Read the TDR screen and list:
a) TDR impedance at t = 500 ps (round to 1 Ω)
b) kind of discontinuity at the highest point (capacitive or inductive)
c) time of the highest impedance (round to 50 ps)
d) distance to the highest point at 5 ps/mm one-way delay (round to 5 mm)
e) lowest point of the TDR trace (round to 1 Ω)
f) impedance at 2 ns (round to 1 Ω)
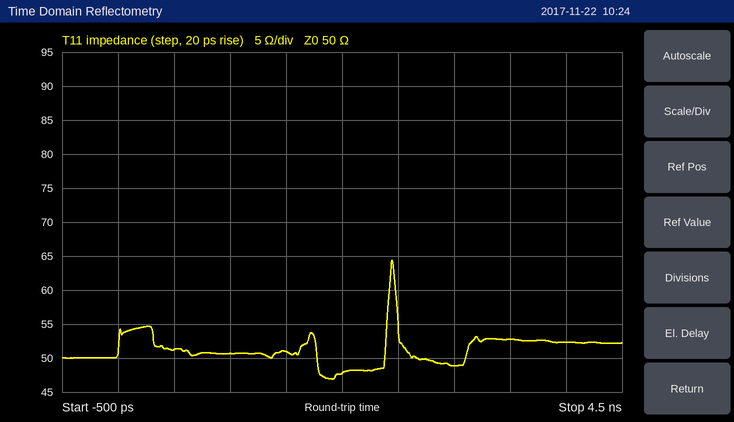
51 Ω
inductive
2.45 ns
245 mm
47 Ω
48 Ω
